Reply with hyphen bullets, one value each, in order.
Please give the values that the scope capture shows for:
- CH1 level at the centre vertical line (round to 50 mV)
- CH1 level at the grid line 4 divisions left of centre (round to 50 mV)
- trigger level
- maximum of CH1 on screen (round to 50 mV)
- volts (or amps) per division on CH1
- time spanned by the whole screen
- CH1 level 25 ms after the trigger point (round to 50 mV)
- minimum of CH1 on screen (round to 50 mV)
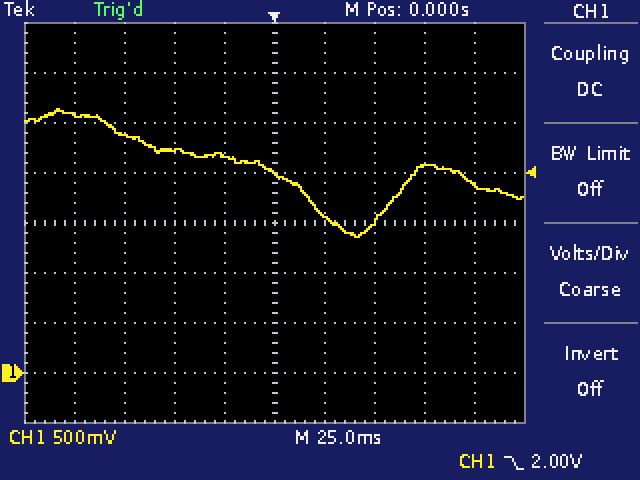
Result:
- 2.00 V
- 2.60 V
- 2.00 V
- 2.65 V
- 500 mV
- 250 ms
- 1.55 V
- 1.35 V
